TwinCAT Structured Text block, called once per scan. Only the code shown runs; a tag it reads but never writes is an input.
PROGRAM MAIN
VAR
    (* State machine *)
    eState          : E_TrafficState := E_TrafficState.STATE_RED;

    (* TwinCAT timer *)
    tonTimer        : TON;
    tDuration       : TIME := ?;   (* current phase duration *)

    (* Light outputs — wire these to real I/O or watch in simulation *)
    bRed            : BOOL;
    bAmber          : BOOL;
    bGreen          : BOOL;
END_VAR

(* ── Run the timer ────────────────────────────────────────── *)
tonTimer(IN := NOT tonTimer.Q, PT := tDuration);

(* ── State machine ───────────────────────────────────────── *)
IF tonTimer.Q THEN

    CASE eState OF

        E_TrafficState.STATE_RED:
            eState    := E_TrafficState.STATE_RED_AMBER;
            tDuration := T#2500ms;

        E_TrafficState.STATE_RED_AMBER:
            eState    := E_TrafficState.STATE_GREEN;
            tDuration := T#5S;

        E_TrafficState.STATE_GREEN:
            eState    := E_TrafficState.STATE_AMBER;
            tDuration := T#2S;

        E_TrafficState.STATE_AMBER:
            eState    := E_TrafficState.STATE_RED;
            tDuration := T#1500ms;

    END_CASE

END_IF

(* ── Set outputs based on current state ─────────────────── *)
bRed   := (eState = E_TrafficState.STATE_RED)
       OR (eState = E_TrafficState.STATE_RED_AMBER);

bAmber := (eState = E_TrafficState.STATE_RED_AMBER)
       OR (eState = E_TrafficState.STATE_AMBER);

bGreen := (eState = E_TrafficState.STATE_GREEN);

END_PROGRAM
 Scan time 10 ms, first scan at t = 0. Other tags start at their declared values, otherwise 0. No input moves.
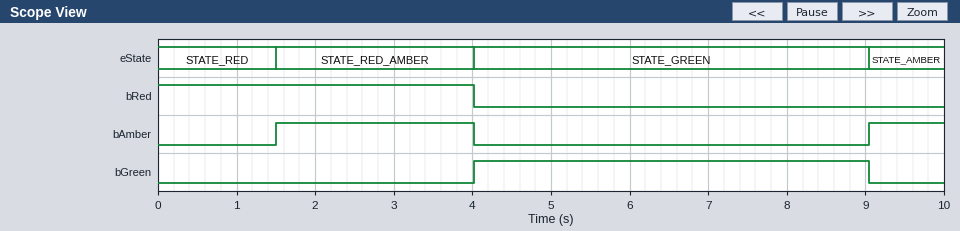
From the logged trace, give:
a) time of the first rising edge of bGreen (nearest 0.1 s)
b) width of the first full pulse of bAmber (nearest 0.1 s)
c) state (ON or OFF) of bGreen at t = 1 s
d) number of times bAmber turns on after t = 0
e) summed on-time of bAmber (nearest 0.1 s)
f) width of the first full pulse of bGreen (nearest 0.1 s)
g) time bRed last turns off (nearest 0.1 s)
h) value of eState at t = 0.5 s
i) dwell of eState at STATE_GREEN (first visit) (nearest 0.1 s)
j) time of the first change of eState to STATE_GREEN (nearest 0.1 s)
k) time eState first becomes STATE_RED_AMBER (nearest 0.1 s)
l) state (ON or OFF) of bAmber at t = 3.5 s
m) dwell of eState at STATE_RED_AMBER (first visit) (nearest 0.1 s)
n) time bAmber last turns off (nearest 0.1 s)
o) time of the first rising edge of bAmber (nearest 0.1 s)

4.0 s
2.5 s
OFF
2
3.5 s
5.0 s
4.0 s
STATE_RED
5.0 s
4.0 s
1.5 s
ON
2.5 s
4.0 s
1.5 s
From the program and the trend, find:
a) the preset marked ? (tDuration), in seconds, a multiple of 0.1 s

1.5 s
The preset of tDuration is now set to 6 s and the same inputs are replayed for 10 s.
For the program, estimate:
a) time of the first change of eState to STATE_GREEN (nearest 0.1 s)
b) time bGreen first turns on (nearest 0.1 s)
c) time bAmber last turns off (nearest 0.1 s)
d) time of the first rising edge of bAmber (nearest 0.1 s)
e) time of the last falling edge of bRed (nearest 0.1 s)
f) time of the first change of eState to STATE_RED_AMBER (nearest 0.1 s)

8.5 s
8.5 s
8.5 s
6.0 s
8.5 s
6.0 s
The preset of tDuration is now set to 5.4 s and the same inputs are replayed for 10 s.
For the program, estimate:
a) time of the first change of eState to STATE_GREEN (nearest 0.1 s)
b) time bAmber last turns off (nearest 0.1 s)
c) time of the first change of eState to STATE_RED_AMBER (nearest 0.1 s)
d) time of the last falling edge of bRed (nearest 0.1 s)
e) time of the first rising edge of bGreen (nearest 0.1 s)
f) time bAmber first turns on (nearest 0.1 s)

7.9 s
7.9 s
5.4 s
7.9 s
7.9 s
5.4 s
